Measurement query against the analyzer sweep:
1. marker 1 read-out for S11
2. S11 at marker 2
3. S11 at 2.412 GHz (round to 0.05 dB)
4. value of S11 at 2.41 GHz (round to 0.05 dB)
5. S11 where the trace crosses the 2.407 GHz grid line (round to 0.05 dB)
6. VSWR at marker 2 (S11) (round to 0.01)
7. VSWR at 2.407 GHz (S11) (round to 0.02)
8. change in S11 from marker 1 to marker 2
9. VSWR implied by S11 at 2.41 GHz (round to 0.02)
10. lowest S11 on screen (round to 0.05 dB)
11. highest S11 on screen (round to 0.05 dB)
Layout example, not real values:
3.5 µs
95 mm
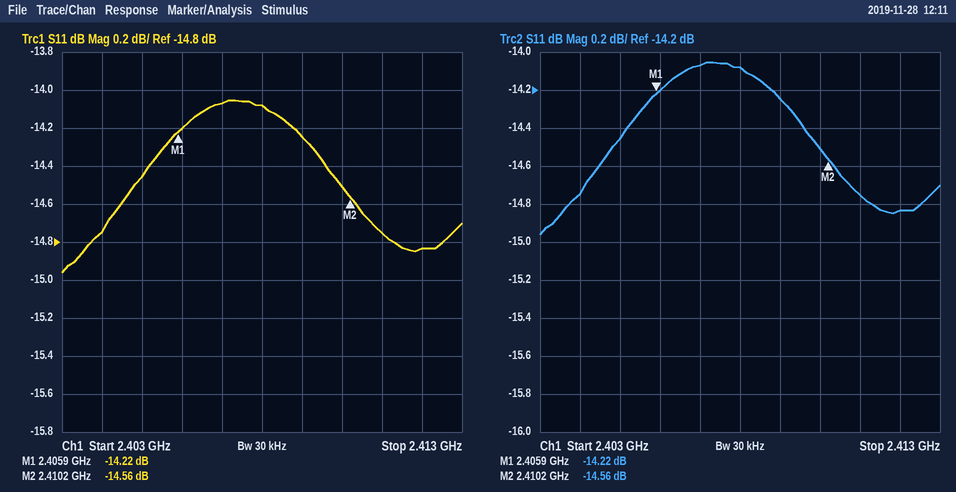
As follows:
-14.22 dB
-14.56 dB
-14.85 dB
-14.50 dB
-14.05 dB
1.46
1.50
-0.34 dB
1.46
-14.95 dB
-14.05 dB
